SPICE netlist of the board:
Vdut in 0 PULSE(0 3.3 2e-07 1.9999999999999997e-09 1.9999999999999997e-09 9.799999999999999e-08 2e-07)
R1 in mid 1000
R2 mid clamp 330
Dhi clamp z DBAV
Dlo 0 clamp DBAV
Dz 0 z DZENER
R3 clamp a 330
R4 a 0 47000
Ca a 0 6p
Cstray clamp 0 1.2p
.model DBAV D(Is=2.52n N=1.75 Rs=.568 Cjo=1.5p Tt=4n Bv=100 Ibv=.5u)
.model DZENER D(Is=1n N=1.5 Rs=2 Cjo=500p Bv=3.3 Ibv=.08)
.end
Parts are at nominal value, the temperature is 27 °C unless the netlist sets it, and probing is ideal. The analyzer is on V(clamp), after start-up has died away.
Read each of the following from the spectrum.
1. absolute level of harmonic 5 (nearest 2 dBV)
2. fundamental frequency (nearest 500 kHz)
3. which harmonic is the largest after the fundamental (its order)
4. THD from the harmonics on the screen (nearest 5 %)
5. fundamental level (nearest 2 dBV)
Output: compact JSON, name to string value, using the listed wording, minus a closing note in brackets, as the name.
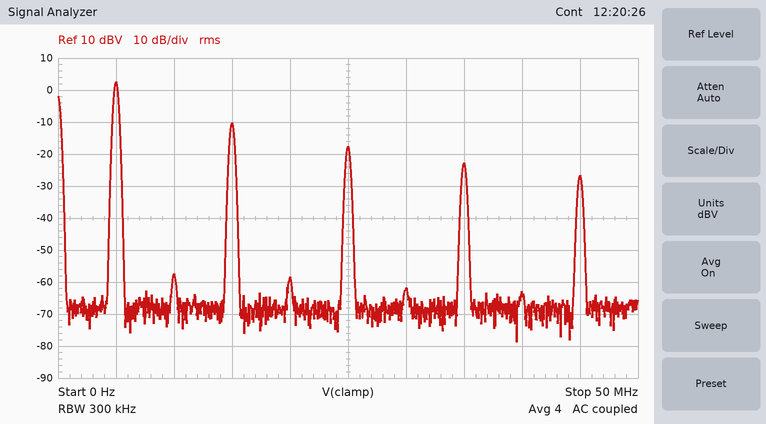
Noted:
{"absolute level of harmonic 5": "-18 dBV", "fundamental frequency": "5.0 MHz", "which harmonic is the largest after the fundamental": "3", "THD from the harmonics on the screen": "25 %", "fundamental level": "2 dBV"}
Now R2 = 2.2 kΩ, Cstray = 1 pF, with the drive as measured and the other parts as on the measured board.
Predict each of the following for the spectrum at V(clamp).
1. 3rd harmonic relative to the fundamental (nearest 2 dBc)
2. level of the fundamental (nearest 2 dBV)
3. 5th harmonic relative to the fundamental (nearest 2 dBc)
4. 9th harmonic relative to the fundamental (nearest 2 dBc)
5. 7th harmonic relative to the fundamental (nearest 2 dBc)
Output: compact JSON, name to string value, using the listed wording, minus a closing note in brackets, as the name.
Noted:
{"3rd harmonic relative to the fundamental": "-16 dBc", "level of the fundamental": "0 dBV", "5th harmonic relative to the fundamental": "-24 dBc", "9th harmonic relative to the fundamental": "-34 dBc", "7th harmonic relative to the fundamental": "-30 dBc"}
